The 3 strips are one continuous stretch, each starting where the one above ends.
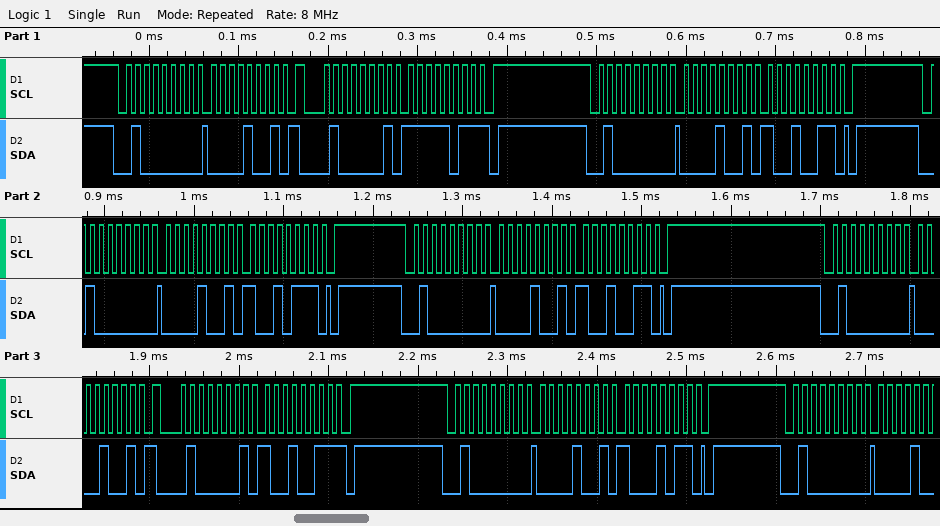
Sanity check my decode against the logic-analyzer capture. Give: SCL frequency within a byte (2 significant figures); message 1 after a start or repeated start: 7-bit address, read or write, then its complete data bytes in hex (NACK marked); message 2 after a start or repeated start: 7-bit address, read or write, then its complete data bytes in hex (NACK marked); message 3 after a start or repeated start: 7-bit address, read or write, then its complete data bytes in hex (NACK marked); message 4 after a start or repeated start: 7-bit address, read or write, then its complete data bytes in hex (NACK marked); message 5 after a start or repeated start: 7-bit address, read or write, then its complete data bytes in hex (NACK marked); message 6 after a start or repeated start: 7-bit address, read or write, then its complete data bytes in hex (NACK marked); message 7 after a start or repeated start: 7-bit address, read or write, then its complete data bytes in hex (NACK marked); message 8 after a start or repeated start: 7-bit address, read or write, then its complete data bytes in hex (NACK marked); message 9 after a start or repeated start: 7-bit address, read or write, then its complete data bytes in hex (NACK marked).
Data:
100 kHz
0x20 write: 09
0x20 read: FB NACK
0x20 write: 09 93
0x20 write: 09 97
0x20 write: 09 93
0x20 write: 09
0x20 read: 93 NACK
0x20 write: 09 8B
0x20 write
